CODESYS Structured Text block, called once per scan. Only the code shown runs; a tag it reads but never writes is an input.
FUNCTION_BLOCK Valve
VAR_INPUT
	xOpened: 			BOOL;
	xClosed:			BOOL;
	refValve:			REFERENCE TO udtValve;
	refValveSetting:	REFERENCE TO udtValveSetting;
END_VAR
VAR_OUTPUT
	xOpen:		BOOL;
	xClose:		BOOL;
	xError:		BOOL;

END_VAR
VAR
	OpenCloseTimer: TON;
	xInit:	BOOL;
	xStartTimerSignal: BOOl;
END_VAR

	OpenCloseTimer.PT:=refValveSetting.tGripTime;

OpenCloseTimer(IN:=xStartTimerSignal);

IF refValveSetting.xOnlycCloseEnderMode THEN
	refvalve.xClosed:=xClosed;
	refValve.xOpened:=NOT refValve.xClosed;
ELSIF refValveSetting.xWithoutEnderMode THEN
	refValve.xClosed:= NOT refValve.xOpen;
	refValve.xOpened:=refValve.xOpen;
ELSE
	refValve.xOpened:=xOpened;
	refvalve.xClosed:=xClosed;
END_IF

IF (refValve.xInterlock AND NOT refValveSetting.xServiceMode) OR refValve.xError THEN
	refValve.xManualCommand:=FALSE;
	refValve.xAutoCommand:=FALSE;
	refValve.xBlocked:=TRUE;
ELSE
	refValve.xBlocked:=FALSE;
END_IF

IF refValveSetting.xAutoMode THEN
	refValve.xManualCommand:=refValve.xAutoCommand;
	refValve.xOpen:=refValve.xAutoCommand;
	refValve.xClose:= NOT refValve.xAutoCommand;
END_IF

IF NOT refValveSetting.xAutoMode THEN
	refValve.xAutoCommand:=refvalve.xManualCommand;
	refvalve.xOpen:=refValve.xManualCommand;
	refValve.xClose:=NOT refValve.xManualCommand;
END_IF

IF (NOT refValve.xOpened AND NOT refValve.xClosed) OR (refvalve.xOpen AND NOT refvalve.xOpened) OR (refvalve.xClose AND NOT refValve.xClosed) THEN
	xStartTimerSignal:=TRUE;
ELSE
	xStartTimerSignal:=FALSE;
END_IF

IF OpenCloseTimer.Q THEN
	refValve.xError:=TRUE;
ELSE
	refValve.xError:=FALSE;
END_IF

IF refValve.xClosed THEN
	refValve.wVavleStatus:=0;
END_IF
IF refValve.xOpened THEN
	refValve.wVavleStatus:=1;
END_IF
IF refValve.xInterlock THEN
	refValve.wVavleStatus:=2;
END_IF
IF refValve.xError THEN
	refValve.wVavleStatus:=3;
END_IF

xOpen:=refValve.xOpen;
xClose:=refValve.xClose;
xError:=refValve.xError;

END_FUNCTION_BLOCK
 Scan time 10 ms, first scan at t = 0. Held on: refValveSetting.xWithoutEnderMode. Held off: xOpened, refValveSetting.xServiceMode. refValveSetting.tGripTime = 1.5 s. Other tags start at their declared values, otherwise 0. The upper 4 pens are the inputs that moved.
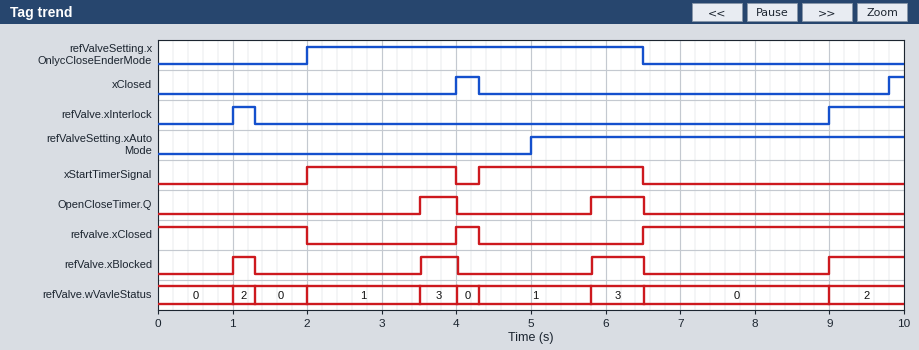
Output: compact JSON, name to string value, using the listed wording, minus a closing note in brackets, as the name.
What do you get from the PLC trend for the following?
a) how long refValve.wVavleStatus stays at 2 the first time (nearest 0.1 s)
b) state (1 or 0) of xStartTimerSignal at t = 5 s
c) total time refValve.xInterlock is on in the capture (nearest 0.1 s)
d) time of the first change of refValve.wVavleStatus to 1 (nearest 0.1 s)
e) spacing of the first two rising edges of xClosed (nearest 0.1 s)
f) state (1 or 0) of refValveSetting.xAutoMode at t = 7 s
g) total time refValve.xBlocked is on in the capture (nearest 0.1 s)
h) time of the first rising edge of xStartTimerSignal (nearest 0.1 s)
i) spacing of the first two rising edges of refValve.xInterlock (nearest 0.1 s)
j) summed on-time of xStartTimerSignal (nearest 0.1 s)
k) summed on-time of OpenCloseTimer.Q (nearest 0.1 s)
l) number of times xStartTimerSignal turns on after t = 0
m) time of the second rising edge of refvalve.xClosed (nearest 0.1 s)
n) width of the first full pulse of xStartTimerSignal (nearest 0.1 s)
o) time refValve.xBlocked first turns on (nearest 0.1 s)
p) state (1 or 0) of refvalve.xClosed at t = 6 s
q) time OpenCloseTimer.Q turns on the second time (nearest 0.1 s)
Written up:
{"how long refValve.wVavleStatus stays at 2 the first time": "0.3 s", "state (1 or 0) of xStartTimerSignal at t = 5 s": "1", "total time refValve.xInterlock is on in the capture": "1.3 s", "time of the first change of refValve.wVavleStatus to 1": "2.0 s", "spacing of the first two rising edges of xClosed": "5.8 s", "state (1 or 0) of refValveSetting.xAutoMode at t = 7 s": "1", "total time refValve.xBlocked is on in the capture": "2.5 s", "time of the first rising edge of xStartTimerSignal": "2.0 s", "spacing of the first two rising edges of refValve.xInterlock": "8.0 s", "summed on-time of xStartTimerSignal": "4.2 s", "summed on-time of OpenCloseTimer.Q": "1.2 s", "number of times xStartTimerSignal turns on after t = 0": "2", "time of the second rising edge of refvalve.xClosed": "6.5 s", "width of the first full pulse of xStartTimerSignal": "2.0 s", "time refValve.xBlocked first turns on": "1.0 s", "state (1 or 0) of refvalve.xClosed at t = 6 s": "0", "time OpenCloseTimer.Q turns on the second time": "5.8 s"}
